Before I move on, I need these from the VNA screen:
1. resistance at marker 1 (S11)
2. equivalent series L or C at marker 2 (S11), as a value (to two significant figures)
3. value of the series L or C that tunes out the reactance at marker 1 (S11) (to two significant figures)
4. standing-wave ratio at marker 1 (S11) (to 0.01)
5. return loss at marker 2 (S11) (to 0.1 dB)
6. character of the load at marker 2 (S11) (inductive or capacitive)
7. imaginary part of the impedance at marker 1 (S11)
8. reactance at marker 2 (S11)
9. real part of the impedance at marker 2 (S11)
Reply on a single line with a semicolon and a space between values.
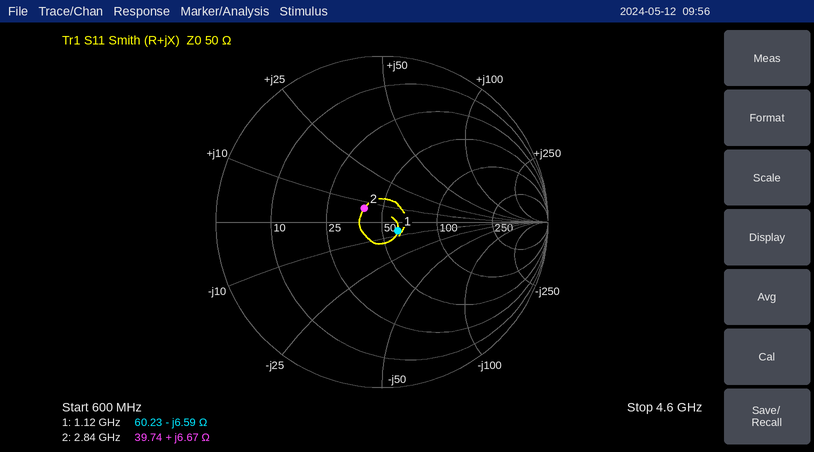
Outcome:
60.23 Ω; 370 pH; 940 pH; 1.25; 17.3 dB; inductive; -6.59 Ω; +6.67 Ω; 39.74 Ω
